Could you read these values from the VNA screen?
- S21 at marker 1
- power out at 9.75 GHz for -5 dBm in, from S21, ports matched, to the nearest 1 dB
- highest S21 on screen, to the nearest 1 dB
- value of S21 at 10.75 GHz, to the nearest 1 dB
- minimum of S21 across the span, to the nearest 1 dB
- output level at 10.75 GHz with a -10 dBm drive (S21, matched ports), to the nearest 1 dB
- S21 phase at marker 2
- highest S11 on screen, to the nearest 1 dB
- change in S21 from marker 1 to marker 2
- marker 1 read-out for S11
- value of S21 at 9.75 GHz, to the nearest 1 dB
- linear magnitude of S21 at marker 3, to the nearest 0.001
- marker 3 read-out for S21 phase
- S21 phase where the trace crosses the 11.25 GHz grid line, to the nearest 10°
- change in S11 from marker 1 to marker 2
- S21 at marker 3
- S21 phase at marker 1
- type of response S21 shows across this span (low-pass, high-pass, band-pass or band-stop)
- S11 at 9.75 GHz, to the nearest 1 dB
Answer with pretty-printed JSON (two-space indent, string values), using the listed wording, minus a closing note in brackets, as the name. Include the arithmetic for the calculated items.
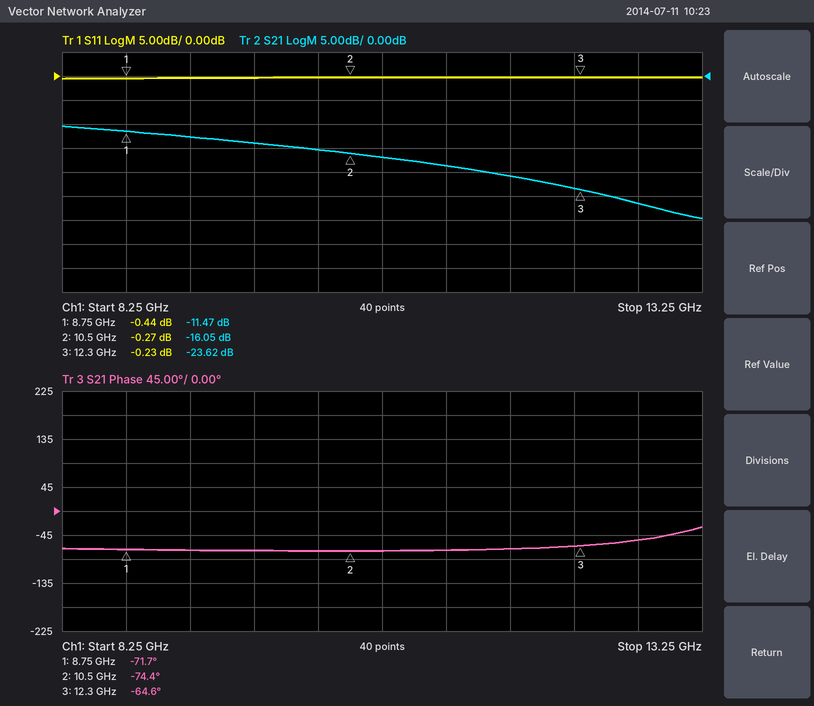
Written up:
{
  "S21 at marker 1": "-11.47 dB",
  "power out at 9.75 GHz for -5 dBm in, from S21, ports matched, to the nearest 1 dB": "-5 dBm + (-14 dB) = -19 dBm",
  "highest S21 on screen, to the nearest 1 dB": "-10 dB",
  "value of S21 at 10.75 GHz, to the nearest 1 dB": "-17 dB",
  "minimum of S21 across the span, to the nearest 1 dB": "-30 dB",
  "output level at 10.75 GHz with a -10 dBm drive (S21, matched ports), to the nearest 1 dB": "-10 dBm + (-17 dB) = -27 dBm",
  "S21 phase at marker 2": "-74.4°",
  "highest S11 on screen, to the nearest 1 dB": "0 dB",
  "change in S21 from marker 1 to marker 2": "-16.05 − (-11.47) = -4.58 dB",
  "marker 1 read-out for S11": "-0.44 dB",
  "value of S21 at 9.75 GHz, to the nearest 1 dB": "-14 dB",
  "linear magnitude of S21 at marker 3, to the nearest 0.001": "10^(-23.62/20) ≈ 0.066",
  "marker 3 read-out for S21 phase": "-64.6°",
  "S21 phase where the trace crosses the 11.25 GHz grid line, to the nearest 10°": "-70°",
  "change in S11 from marker 1 to marker 2": "-0.27 − (-0.44) = 0.17 dB",
  "S21 at marker 3": "-23.62 dB",
  "S21 phase at marker 1": "-71.7°",
  "type of response S21 shows across this span": "low-pass",
  "S11 at 9.75 GHz, to the nearest 1 dB": "0 dB"
}
